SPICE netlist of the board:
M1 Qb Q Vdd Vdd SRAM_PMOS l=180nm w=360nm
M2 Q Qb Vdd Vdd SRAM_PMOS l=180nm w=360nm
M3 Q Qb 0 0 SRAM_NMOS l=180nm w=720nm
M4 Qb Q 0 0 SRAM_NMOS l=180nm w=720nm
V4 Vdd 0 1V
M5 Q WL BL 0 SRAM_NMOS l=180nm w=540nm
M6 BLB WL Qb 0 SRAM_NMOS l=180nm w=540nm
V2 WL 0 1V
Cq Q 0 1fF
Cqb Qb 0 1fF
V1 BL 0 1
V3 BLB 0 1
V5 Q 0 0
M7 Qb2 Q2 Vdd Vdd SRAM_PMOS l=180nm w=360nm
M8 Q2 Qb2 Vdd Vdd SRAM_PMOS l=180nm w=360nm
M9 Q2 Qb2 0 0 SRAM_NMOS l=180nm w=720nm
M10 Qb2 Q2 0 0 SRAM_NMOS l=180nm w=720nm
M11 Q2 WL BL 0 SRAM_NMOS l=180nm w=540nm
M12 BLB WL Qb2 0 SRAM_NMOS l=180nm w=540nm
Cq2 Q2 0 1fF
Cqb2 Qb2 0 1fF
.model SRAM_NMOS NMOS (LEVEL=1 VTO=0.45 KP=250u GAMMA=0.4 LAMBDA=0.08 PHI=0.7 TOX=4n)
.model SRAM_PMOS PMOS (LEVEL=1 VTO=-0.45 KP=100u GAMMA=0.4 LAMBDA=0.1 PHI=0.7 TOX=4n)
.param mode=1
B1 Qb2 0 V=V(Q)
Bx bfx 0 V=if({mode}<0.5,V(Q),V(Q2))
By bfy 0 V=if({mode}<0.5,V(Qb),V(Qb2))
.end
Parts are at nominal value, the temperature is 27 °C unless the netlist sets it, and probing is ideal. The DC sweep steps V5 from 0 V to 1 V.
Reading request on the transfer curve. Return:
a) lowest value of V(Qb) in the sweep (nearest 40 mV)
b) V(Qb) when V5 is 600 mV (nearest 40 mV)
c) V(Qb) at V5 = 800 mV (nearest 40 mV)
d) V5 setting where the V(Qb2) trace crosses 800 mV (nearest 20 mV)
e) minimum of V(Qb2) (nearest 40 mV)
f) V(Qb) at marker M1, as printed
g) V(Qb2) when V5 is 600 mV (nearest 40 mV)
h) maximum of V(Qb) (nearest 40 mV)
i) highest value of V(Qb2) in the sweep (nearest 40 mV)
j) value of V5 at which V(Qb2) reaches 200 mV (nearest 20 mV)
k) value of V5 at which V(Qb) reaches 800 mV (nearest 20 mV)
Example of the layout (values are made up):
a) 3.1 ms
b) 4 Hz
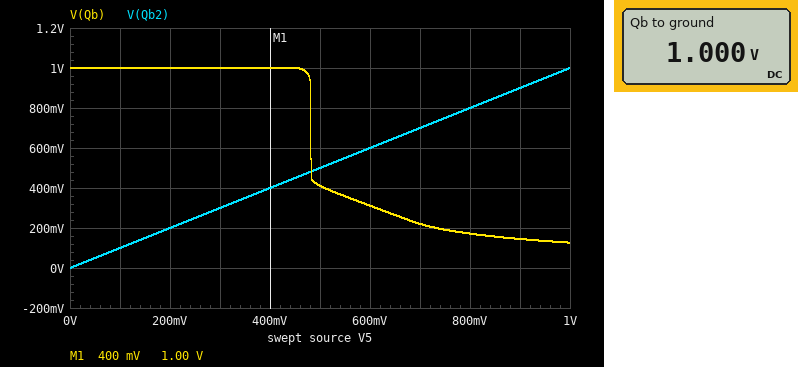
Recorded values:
a) 120 mV
b) 320 mV
c) 160 mV
d) 800 mV
e) 0 V
f) 1.00 V
g) 600 mV
h) 1.00 V
i) 1.00 V
j) 200 mV
k) 480 mV
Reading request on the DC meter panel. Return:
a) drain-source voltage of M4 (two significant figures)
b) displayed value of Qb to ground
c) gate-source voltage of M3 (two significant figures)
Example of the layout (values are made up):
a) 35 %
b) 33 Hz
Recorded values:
a) 1.0 V
b) 1.000 V
c) 1.0 V
